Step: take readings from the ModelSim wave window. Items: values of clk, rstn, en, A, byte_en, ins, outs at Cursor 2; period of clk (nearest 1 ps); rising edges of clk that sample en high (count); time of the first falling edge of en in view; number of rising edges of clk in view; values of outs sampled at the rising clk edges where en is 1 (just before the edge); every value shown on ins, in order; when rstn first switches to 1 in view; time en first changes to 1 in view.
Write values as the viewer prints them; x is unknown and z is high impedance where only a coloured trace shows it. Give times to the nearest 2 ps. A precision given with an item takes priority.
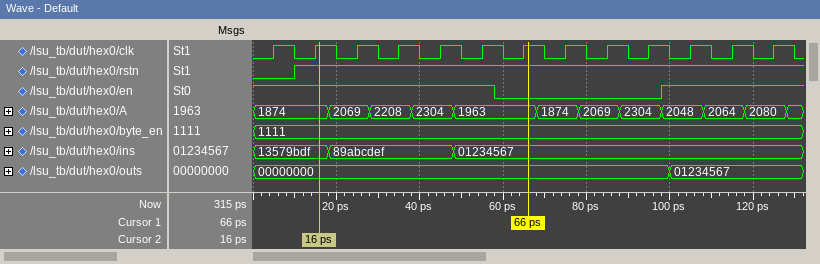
clk=1, rstn=1, en=1, A=1874, byte_en=1111, ins=13579bdf, outs=00000000
10 ps
9
58 ps
13
00000000, 00000000, 00000000, 00000000, 00000000, 00000000, 01234567, 01234567, 01234567
13579bdf, 89abcdef, 01234567
10 ps
98 ps
